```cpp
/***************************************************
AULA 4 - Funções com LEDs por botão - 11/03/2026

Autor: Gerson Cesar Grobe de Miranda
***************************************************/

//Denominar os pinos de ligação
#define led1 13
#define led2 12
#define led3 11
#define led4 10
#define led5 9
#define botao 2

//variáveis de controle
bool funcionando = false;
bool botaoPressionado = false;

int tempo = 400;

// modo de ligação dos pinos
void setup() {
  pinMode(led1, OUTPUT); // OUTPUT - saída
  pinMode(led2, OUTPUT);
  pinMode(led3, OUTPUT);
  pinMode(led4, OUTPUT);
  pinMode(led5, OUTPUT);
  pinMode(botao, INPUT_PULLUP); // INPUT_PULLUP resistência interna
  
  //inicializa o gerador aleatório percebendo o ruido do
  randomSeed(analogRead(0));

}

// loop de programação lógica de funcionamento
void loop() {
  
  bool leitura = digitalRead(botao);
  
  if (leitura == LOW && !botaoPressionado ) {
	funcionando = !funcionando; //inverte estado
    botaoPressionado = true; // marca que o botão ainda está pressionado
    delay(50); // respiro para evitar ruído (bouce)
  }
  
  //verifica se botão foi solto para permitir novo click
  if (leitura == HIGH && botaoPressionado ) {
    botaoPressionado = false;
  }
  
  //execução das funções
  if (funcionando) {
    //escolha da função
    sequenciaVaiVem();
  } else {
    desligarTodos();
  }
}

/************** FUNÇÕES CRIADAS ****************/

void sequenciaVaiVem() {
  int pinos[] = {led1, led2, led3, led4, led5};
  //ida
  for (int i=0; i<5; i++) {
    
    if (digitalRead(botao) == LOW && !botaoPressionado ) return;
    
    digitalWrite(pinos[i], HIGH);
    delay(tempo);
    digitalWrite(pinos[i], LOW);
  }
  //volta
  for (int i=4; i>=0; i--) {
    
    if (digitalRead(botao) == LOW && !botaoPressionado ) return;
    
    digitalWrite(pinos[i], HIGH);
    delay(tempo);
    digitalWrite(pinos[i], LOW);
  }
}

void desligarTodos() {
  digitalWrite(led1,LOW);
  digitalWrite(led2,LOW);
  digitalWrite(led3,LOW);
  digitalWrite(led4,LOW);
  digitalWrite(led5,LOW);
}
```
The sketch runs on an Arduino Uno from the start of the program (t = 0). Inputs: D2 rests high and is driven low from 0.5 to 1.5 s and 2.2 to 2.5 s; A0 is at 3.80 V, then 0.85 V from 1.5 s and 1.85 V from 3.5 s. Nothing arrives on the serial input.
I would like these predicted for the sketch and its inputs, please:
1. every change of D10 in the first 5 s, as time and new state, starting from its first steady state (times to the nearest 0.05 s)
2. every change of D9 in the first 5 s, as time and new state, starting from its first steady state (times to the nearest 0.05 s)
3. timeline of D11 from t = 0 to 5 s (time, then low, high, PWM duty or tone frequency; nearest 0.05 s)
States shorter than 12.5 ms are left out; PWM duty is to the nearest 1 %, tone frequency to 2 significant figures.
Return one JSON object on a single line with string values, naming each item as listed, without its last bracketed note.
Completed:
{"every change of D10 in the first 5 s, as time and new state, starting from its first steady state": "0 s low; 1.75 s high; 2.15 s low; 2.95 s high; 3.35 s low", "every change of D9 in the first 5 s, as time and new state, starting from its first steady state": "0 s low; 2.15 s high; 2.95 s low", "timeline of D11 from t = 0 to 5 s": "0 s low; 1.35 s high; 1.75 s low; 3.35 s high; 3.75 s low"}
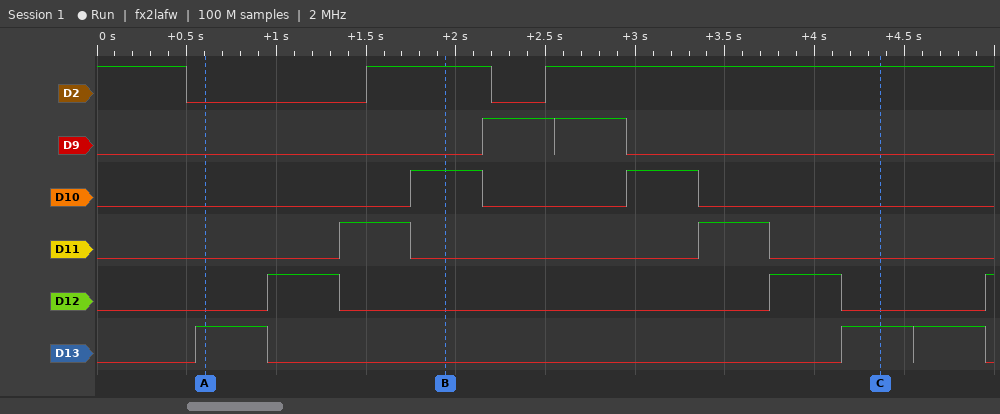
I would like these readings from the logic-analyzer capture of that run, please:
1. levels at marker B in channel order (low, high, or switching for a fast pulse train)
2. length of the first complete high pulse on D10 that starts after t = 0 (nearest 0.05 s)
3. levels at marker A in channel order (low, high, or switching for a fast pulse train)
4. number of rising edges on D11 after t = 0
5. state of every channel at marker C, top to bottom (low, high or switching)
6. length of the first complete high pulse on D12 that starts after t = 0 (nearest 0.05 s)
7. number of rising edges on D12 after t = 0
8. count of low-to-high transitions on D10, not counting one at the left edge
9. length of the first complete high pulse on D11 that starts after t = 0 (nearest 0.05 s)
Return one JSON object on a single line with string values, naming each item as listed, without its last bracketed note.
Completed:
{"levels at marker B in channel order": "D2 high, D9 low, D10 high, D11 low, D12 low, D13 low", "length of the first complete high pulse on D10 that starts after t = 0": "0.40 s", "levels at marker A in channel order": "D2 low, D9 low, D10 low, D11 low, D12 low, D13 high", "number of rising edges on D11 after t = 0": "2", "state of every channel at marker C, top to bottom": "D2 high, D9 low, D10 low, D11 low, D12 low, D13 high", "length of the first complete high pulse on D12 that starts after t = 0": "0.40 s", "number of rising edges on D12 after t = 0": "3", "count of low-to-high transitions on D10, not counting one at the left edge": "2", "length of the first complete high pulse on D11 that starts after t = 0": "0.40 s"}
